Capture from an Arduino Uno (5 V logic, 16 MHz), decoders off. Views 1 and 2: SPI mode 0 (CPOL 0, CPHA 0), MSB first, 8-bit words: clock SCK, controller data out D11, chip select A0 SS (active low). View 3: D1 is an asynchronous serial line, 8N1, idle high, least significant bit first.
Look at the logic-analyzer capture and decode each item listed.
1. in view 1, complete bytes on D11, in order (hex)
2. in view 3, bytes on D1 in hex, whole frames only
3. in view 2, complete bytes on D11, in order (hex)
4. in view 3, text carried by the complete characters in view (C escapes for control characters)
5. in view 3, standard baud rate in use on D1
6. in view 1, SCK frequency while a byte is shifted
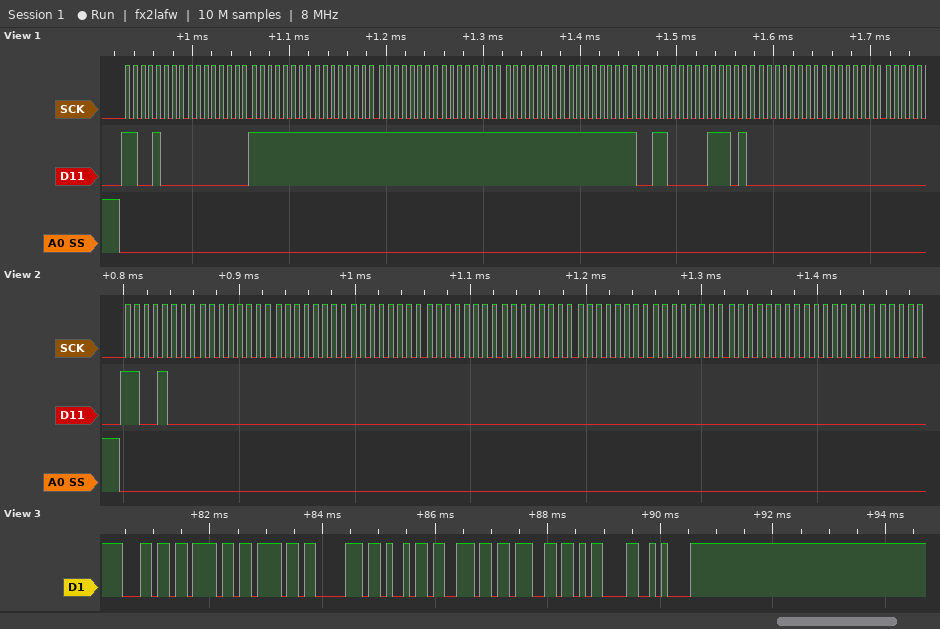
C8 00 FF FF FF FF FF FF 98 3A 00 00
6C 6F 6F 70 69 6E 67 0D 0A
0xC8 0x00 0x00 0x00 0x00 0x00 0x00 0x00 0x00 0x00
"looping\r\n"
9600 baud
125 kHz
